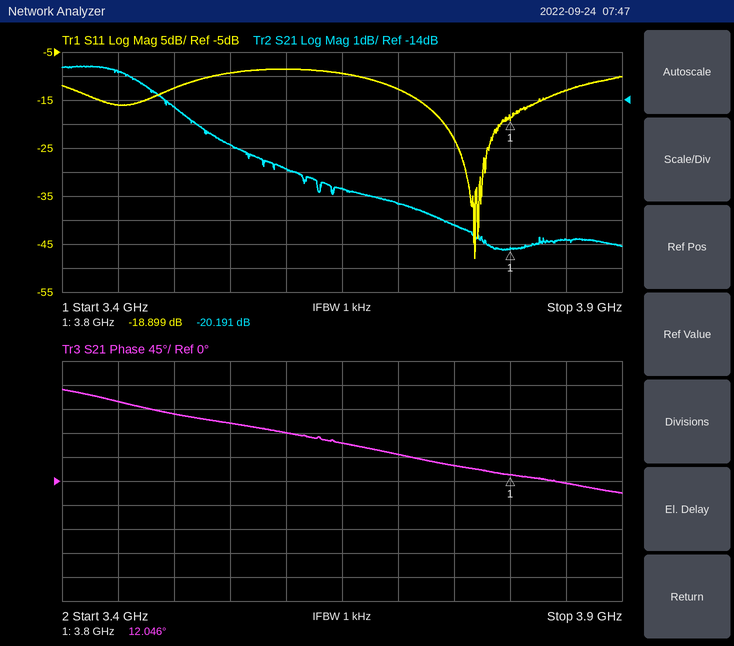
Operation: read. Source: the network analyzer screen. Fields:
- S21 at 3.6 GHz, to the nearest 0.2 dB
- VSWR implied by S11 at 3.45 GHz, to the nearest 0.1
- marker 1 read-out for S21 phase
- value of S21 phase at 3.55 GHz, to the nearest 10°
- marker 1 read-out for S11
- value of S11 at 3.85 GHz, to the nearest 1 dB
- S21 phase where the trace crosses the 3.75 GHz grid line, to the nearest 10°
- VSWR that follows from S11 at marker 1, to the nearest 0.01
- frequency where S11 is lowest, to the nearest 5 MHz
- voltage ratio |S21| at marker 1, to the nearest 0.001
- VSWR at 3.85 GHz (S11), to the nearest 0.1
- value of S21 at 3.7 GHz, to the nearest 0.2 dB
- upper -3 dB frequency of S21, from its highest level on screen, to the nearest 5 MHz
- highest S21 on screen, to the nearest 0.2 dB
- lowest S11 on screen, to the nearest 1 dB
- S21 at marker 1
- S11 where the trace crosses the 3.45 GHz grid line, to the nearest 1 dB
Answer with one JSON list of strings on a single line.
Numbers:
["-16.8 dB", "1.4", "12.046°", "110°", "-18.899 dB", "-13 dB", "30°", "1.26", "3.770 GHz", "0.098", "1.6", "-18.4 dB", "3.540 GHz", "-12.6 dB", "-48 dB", "-20.191 dB", "-16 dB"]
